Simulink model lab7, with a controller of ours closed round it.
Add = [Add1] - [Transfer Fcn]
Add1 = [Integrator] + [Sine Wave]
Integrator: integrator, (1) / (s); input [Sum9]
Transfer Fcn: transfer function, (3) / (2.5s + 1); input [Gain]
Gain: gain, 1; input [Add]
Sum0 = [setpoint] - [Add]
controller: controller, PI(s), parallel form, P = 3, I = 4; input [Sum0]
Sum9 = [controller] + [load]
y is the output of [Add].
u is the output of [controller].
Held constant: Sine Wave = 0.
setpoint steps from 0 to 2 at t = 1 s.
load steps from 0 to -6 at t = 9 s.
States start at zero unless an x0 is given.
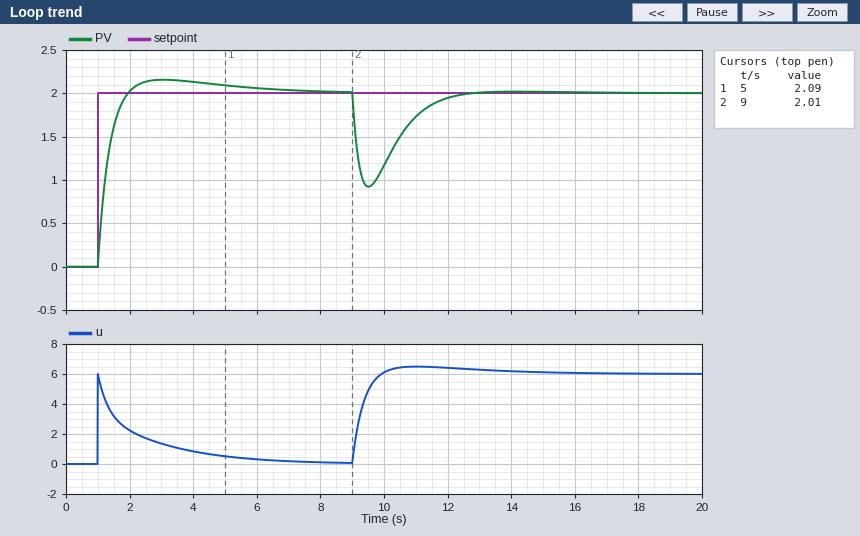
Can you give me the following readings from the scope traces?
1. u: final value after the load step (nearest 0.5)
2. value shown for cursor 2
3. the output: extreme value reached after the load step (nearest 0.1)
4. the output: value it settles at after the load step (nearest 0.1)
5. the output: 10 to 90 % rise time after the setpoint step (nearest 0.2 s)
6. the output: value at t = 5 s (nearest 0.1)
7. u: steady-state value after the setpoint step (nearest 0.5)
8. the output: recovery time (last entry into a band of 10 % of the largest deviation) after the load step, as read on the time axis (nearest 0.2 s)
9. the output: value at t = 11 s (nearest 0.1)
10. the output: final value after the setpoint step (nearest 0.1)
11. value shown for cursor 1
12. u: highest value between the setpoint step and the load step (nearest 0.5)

6.0
2.01
0.9
2.0
0.6 s
2.1
0.0
11.6 s
1.7
2.0
2.09
6.0
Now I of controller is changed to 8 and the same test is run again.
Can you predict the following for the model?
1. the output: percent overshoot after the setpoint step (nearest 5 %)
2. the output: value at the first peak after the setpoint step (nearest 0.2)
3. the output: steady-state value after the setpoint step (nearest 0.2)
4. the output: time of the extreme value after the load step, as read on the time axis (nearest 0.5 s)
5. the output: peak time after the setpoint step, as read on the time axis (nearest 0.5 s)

15 %
2.2
2.0
9.5 s
2.0 s
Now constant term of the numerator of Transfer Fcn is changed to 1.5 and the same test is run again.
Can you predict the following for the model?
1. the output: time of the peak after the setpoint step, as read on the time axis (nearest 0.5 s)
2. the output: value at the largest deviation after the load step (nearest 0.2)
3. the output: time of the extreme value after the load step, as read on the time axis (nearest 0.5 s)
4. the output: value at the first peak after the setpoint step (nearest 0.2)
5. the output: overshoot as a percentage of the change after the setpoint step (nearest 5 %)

2.5 s
0.8
9.5 s
2.2
10 %
